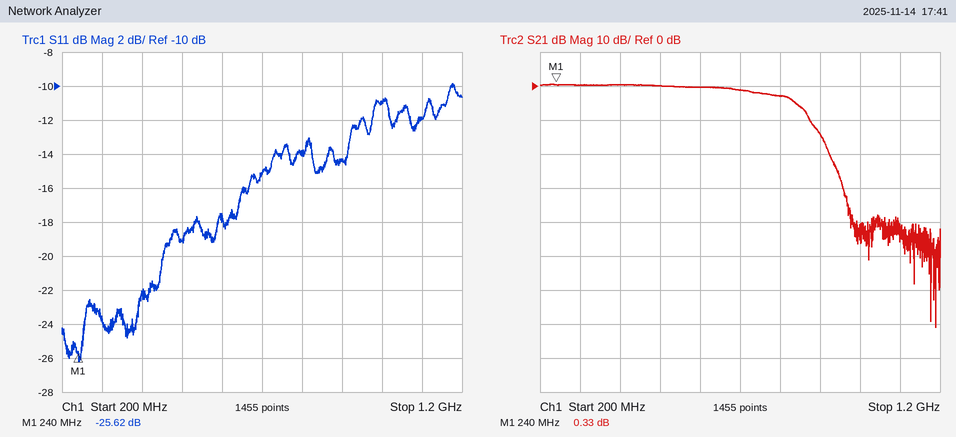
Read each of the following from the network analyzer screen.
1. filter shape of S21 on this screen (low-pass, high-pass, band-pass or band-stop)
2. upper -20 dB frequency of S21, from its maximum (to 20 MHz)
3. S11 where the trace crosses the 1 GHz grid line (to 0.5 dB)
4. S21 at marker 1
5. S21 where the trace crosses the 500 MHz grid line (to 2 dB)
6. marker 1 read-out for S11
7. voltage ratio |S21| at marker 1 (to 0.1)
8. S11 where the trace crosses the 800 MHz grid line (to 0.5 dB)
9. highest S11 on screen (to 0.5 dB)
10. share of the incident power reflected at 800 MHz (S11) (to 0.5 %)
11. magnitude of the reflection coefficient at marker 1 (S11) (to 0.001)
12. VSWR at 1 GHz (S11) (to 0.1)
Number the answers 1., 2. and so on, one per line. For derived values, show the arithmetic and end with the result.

1. low-pass
2. 920 MHz
3. -11.0 dB
4. 0.33 dB
5. 0 dB
6. -25.62 dB
7. 10^(0.33/20) ≈ 1.0
8. -14.0 dB
9. -10.0 dB
10. 10^(-14/10) ≈ 4.0 %
11. 10^(-25.62/20) ≈ 0.052
12. |Γ| = 10^(-11/20) = 0.2818; VSWR = (1 + 0.2818)/(1 − 0.2818) ≈ 1.8
